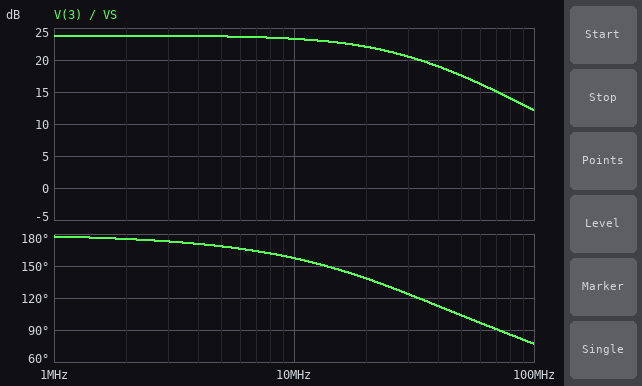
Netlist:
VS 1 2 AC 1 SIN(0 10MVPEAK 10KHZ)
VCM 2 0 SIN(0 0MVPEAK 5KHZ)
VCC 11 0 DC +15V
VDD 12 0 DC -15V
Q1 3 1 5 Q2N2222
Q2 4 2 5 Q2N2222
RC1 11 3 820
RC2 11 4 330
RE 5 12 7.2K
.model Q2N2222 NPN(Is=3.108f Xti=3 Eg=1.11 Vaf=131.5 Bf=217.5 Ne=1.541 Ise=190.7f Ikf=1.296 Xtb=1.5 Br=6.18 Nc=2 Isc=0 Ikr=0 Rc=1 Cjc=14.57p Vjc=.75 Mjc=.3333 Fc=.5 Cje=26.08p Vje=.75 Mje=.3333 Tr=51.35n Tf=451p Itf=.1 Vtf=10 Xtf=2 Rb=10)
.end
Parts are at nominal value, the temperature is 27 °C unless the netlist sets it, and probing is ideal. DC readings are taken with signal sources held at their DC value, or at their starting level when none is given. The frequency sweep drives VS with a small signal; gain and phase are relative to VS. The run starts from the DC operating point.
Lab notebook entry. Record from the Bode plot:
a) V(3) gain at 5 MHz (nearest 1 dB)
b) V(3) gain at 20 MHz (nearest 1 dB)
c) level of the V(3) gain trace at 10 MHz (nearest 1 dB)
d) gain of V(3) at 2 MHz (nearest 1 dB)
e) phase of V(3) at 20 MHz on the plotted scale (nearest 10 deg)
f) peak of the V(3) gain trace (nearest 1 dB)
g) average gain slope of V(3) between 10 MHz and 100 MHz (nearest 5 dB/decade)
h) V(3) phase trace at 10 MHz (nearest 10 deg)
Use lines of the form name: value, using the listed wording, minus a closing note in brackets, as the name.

V(3) gain at 5 MHz: 24 dB
V(3) gain at 20 MHz: 22 dB
level of the V(3) gain trace at 10 MHz: 23 dB
gain of V(3) at 2 MHz: 24 dB
phase of V(3) at 20 MHz on the plotted scale: 140 deg
peak of the V(3) gain trace: 24 dB
average gain slope of V(3) between 10 MHz and 100 MHz: -10 dB/decade
V(3) phase trace at 10 MHz: 160 deg
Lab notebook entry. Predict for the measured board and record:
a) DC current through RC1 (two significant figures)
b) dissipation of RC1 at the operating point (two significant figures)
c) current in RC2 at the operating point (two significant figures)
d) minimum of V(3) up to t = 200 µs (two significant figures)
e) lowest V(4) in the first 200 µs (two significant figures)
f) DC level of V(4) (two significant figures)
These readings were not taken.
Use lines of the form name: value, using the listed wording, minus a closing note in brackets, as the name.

DC current through RC1: 980 µA
dissipation of RC1 at the operating point: 790 µW
current in RC2 at the operating point: 990 µA
minimum of V(3) up to t = 200 µs: 14 V
lowest V(4) in the first 200 µs: 15 V
DC level of V(4): 15 V
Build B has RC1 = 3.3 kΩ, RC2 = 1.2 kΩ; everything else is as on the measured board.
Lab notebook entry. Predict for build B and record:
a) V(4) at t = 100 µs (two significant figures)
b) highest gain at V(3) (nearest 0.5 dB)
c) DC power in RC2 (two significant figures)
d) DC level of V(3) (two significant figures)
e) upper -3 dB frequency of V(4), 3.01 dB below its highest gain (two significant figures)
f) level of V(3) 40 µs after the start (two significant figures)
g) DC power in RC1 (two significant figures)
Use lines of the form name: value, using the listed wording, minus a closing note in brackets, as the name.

V(4) at t = 100 µs: 14 V
highest gain at V(3): 36.0 dB
DC power in RC2: 1.2 mW
DC level of V(3): 12 V
upper -3 dB frequency of V(4), 3.01 dB below its highest gain: 15 MHz
level of V(3) 40 µs after the start: 11 V
DC power in RC1: 3.2 mW
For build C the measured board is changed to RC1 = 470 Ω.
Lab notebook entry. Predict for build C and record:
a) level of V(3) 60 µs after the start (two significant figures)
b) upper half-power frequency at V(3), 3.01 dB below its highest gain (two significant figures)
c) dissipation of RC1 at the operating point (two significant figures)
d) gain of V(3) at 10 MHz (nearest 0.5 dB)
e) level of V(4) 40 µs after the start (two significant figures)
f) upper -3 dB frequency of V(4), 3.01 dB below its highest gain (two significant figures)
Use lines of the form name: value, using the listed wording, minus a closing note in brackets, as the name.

level of V(3) 60 µs after the start: 15 V
upper half-power frequency at V(3), 3.01 dB below its highest gain: 46 MHz
dissipation of RC1 at the operating point: 460 µW
gain of V(3) at 10 MHz: 19.0 dB
level of V(4) 40 µs after the start: 15 V
upper -3 dB frequency of V(4), 3.01 dB below its highest gain: 53 MHz
